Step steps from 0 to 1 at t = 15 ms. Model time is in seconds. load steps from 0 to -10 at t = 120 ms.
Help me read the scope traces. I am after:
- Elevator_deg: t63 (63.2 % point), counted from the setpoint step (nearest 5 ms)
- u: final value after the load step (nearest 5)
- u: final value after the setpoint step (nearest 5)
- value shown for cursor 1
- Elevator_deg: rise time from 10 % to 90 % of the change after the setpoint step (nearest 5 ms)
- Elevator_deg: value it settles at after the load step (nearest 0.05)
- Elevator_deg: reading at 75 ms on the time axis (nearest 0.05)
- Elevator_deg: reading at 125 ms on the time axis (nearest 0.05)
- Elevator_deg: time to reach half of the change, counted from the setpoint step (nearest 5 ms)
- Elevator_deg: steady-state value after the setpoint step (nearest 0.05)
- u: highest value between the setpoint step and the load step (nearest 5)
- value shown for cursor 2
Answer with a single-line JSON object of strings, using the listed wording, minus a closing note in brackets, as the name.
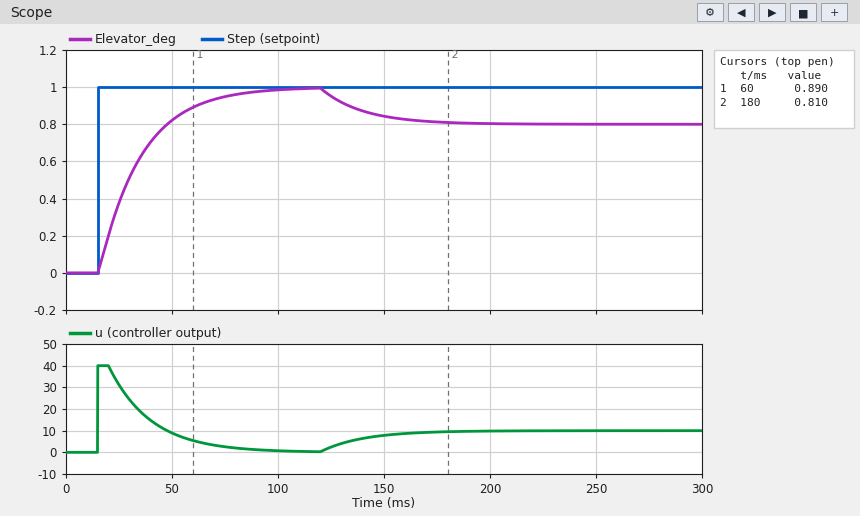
{"Elevator_deg: t63 (63.2 % point), counted from the setpoint step": "20 ms", "u: final value after the load step": "10", "u: final value after the setpoint step": "0", "value shown for cursor 1": "0.890", "Elevator_deg: rise time from 10 % to 90 % of the change after the setpoint step": "45 ms", "Elevator_deg: value it settles at after the load step": "0.80", "Elevator_deg: reading at 75 ms on the time axis": "0.95", "Elevator_deg: reading at 125 ms on the time axis": "0.95", "Elevator_deg: time to reach half of the change, counted from the setpoint step": "15 ms", "Elevator_deg: steady-state value after the setpoint step": "1.00", "u: highest value between the setpoint step and the load step": "40", "value shown for cursor 2": "0.810"}
